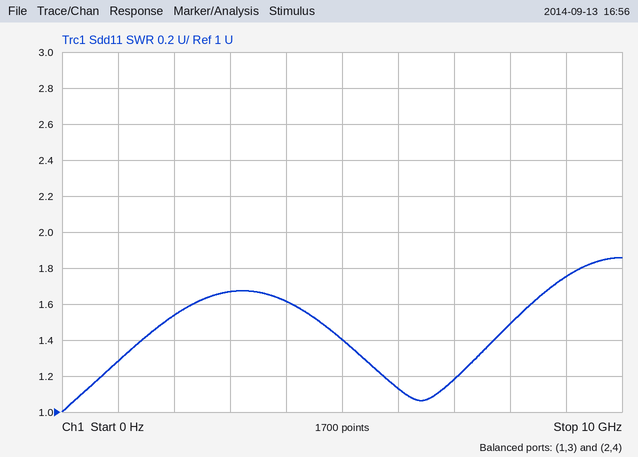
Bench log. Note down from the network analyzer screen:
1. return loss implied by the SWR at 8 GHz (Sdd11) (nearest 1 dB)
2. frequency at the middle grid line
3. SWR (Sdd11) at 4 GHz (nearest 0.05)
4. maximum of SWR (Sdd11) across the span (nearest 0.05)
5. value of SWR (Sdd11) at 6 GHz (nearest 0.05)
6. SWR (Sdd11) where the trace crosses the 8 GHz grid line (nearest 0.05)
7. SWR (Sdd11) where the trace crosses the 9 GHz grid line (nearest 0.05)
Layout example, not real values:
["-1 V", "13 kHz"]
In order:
["14 dB", "5 GHz", "1.60", "1.85", "1.15", "1.50", "1.75"]
